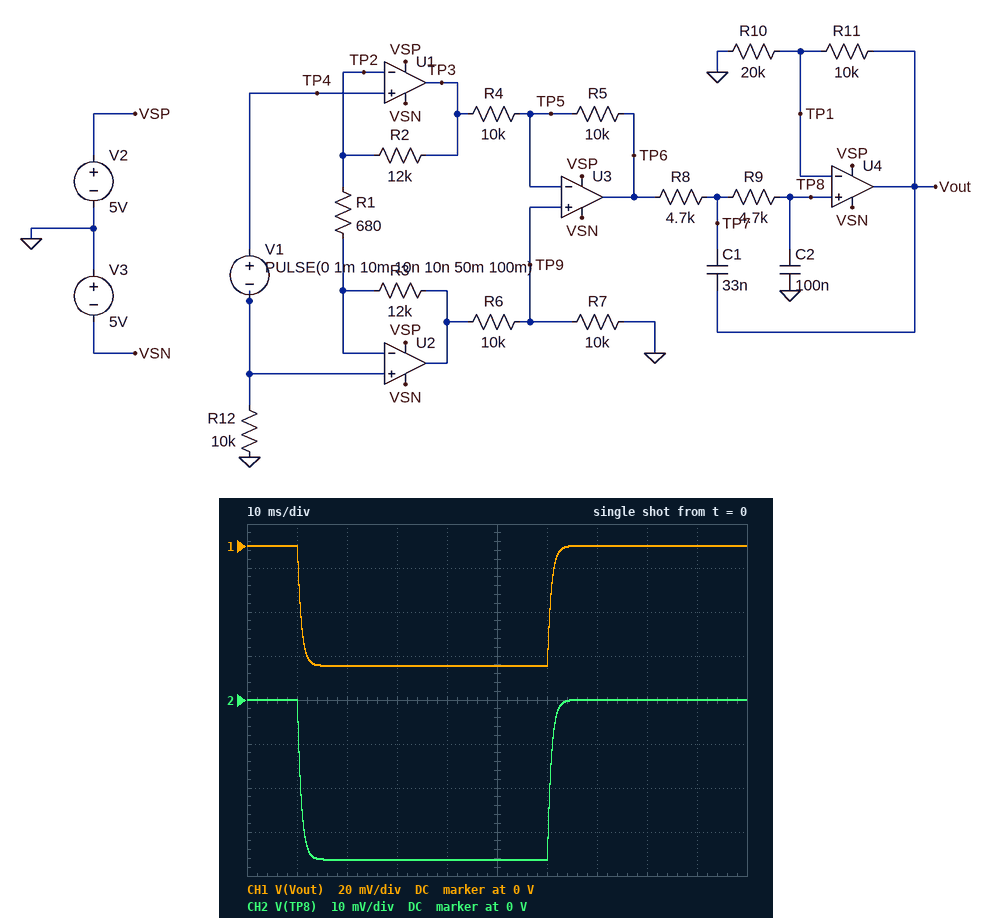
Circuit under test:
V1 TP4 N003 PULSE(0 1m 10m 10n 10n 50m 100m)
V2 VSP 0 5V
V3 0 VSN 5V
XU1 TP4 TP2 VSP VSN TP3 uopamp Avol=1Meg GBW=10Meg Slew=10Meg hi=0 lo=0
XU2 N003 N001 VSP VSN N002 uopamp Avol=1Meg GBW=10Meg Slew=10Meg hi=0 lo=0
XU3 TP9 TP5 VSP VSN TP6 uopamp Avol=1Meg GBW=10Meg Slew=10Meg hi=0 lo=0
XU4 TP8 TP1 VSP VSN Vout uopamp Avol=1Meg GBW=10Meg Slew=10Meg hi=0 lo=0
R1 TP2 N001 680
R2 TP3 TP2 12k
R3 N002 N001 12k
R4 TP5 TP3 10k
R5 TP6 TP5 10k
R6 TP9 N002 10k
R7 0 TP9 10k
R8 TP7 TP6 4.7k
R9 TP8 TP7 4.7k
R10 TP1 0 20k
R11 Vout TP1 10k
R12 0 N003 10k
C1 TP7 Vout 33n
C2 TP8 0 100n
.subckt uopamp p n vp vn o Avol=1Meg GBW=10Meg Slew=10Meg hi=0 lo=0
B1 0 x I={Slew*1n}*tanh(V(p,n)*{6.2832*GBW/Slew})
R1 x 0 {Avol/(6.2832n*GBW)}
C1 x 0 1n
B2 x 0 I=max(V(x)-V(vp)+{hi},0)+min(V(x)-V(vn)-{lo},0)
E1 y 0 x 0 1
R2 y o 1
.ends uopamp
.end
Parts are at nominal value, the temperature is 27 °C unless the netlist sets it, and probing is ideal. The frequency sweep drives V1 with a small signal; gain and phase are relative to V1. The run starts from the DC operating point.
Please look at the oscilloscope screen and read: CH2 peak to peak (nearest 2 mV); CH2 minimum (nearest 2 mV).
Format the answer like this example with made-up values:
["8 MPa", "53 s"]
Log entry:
["36 mV", "-36 mV"]
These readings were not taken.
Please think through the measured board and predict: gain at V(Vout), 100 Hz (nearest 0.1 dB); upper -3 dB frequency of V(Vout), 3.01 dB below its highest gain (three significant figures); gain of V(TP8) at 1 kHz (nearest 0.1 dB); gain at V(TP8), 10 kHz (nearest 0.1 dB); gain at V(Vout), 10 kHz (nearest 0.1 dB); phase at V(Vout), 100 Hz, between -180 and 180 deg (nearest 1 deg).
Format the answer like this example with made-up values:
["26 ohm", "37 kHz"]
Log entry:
["33.8 dB", "204 Hz", "16.0 dB", "-18.1 dB", "-14.6 dB", "151 deg"]
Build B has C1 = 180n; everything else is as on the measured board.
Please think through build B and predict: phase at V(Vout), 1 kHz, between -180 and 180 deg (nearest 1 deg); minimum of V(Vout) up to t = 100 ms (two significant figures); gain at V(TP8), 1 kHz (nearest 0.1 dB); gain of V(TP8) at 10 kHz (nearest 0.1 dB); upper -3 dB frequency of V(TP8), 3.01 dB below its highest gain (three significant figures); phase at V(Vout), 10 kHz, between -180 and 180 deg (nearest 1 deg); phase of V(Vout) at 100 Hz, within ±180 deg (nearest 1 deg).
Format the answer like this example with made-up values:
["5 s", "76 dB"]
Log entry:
["12 deg", "-68 mV", "7.6 dB", "-32.7 dB", "300 Hz", "-1 deg", "159 deg"]
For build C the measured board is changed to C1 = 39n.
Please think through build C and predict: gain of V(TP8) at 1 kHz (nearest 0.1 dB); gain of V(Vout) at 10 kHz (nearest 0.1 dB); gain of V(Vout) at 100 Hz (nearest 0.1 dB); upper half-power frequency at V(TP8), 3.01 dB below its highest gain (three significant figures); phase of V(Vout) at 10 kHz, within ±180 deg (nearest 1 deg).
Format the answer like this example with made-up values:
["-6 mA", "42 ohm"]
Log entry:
["15.9 dB", "-16.0 dB", "33.9 dB", "213 Hz", "7 deg"]
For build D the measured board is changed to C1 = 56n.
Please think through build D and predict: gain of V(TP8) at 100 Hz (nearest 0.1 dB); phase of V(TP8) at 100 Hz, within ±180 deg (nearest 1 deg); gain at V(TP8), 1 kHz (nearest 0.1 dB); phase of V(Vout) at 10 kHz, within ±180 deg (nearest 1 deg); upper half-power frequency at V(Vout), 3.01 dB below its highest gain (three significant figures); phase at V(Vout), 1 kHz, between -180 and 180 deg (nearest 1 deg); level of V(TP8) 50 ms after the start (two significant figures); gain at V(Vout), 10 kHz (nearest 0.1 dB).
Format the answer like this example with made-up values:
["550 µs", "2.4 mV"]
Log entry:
["30.5 dB", "152 deg", "15.1 dB", "4 deg", "240 Hz", "52 deg", "-36 mV", "-19.1 dB"]
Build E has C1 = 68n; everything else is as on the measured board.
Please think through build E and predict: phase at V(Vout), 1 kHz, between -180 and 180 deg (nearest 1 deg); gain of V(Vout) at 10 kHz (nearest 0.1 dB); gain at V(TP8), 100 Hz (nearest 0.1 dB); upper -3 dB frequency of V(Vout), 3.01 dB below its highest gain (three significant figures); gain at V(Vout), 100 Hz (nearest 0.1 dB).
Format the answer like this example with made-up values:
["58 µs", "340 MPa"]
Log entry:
["45 deg", "-20.8 dB", "30.7 dB", "262 Hz", "34.2 dB"]
